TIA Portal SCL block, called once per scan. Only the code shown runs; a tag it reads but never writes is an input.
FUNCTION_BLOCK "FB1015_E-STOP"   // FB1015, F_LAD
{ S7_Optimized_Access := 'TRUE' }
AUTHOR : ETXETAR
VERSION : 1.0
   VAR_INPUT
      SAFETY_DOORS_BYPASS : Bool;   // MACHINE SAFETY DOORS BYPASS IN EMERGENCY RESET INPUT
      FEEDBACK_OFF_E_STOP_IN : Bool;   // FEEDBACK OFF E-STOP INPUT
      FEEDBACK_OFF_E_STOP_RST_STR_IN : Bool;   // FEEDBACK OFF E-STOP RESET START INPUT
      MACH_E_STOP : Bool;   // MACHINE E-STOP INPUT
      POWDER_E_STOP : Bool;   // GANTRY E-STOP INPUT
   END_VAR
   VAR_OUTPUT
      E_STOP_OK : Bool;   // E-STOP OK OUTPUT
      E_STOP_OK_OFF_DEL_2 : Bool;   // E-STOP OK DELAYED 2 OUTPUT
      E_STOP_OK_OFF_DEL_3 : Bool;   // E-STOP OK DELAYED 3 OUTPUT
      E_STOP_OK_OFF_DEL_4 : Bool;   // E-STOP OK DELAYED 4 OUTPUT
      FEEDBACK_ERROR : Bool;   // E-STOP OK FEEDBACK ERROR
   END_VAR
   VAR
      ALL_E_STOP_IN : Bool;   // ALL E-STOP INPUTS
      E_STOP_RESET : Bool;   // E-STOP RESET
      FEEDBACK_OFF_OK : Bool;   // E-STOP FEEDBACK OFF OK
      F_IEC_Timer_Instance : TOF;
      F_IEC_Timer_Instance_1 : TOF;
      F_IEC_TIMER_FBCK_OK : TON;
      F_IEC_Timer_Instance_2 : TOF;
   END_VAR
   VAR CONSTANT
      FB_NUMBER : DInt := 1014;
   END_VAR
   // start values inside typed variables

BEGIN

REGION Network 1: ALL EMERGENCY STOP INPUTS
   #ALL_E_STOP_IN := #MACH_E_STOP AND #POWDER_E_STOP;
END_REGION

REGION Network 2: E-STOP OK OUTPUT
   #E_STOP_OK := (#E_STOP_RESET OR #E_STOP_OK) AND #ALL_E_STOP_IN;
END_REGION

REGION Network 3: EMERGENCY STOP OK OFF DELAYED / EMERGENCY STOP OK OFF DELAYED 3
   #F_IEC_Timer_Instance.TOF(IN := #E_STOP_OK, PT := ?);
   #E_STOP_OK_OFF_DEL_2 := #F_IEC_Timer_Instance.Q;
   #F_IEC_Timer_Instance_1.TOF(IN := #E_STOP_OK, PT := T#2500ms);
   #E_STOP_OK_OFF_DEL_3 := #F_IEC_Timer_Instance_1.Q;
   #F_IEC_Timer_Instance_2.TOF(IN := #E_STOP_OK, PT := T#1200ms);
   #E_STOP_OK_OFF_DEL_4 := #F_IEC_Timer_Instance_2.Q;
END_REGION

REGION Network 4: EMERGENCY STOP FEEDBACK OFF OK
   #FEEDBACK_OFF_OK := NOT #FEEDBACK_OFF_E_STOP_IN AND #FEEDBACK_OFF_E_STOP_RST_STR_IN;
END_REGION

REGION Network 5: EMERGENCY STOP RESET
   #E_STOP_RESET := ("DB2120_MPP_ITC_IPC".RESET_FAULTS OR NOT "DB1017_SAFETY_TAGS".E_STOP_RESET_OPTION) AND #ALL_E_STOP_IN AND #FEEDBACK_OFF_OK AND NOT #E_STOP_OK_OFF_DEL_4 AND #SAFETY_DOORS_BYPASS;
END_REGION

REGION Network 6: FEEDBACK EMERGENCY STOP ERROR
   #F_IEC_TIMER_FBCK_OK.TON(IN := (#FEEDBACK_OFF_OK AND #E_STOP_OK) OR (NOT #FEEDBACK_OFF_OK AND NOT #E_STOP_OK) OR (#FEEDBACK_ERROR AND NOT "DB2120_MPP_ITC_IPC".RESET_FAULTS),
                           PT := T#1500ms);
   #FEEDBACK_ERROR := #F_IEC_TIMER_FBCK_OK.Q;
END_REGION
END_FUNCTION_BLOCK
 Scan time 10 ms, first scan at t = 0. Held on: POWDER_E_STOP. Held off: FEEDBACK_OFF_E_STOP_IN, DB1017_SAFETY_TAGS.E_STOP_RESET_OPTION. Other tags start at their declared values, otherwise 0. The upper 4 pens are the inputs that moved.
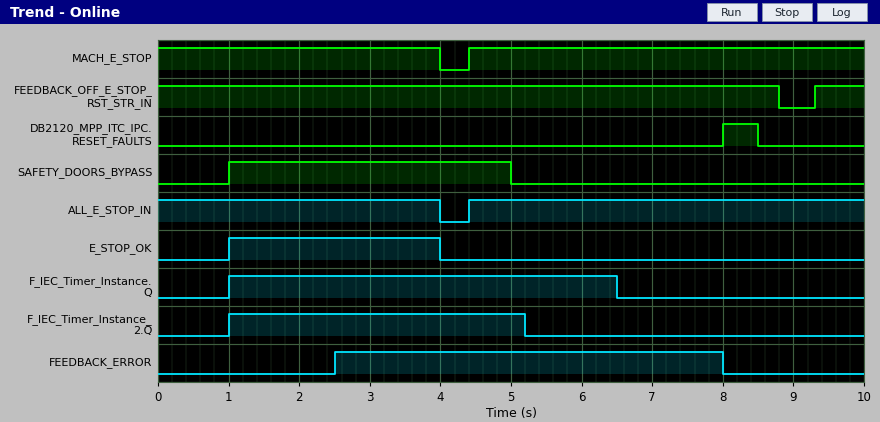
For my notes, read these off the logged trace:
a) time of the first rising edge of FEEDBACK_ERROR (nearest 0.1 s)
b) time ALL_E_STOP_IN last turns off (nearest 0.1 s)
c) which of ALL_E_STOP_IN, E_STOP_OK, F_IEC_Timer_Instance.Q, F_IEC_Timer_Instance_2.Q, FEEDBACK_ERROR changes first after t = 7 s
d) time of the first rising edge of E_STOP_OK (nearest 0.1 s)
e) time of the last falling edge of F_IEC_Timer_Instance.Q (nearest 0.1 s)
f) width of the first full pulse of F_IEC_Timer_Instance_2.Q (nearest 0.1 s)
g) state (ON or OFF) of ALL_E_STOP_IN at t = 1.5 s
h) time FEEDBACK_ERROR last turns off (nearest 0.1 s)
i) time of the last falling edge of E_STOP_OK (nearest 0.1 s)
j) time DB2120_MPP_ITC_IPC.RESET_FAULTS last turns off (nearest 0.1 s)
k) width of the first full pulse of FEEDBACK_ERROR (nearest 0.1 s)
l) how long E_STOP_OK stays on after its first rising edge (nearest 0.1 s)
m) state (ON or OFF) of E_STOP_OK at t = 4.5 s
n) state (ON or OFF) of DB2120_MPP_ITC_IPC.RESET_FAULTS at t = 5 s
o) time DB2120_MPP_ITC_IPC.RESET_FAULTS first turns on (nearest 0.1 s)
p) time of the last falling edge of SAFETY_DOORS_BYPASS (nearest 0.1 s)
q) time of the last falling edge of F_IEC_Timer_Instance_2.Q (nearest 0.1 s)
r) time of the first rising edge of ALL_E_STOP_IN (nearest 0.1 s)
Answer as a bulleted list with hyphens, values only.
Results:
- 2.5 s
- 4.0 s
- FEEDBACK_ERROR
- 1.0 s
- 6.5 s
- 4.2 s
- ON
- 8.0 s
- 4.0 s
- 8.5 s
- 5.5 s
- 3.0 s
- OFF
- OFF
- 8.0 s
- 5.0 s
- 5.2 s
- 4.4 s
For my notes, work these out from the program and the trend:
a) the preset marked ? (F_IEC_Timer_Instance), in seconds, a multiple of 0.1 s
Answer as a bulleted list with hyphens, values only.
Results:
- 2.5 s
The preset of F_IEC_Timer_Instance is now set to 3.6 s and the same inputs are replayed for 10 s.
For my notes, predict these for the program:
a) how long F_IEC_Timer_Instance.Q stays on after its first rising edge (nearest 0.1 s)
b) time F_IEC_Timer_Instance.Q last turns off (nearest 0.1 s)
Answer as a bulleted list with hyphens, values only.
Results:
- 6.6 s
- 7.6 s
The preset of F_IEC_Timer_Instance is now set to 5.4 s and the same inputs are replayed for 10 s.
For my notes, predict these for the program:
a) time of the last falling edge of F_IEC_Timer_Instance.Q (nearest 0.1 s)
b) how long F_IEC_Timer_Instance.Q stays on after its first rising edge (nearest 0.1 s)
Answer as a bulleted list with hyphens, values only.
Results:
- 9.4 s
- 8.4 s
